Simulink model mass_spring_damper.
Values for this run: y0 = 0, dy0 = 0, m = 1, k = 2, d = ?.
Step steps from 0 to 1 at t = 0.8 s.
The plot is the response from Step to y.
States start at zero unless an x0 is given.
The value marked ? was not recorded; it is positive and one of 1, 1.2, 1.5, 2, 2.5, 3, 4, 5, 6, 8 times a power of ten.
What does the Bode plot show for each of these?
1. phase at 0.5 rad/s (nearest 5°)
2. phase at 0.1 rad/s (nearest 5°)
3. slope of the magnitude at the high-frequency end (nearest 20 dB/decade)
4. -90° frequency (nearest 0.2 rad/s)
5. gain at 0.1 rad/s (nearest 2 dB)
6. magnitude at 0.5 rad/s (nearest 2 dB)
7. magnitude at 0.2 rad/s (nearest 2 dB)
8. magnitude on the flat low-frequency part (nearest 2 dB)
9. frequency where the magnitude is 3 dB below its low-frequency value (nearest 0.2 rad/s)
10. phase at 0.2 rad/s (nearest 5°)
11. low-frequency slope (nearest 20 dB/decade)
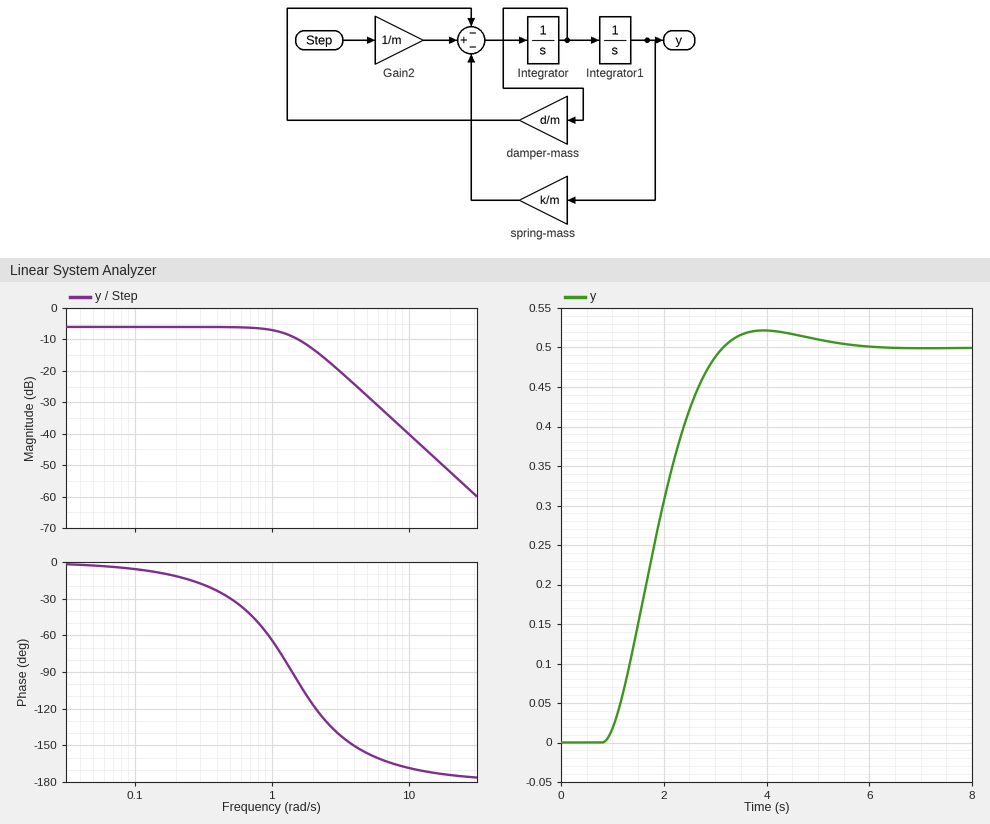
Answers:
-30°
-5°
-40 dB/decade
1.4 rad/s
-6 dB
-6 dB
-6 dB
-6 dB
1.4 rad/s
-10°
0 dB/decade
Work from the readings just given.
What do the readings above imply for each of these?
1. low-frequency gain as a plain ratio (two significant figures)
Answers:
0.50
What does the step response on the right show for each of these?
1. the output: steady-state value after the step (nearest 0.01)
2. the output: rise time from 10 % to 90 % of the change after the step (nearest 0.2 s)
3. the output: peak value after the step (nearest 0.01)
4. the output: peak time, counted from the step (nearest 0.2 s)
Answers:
0.50
1.6 s
0.52
3.2 s
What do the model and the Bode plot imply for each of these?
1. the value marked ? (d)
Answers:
2
